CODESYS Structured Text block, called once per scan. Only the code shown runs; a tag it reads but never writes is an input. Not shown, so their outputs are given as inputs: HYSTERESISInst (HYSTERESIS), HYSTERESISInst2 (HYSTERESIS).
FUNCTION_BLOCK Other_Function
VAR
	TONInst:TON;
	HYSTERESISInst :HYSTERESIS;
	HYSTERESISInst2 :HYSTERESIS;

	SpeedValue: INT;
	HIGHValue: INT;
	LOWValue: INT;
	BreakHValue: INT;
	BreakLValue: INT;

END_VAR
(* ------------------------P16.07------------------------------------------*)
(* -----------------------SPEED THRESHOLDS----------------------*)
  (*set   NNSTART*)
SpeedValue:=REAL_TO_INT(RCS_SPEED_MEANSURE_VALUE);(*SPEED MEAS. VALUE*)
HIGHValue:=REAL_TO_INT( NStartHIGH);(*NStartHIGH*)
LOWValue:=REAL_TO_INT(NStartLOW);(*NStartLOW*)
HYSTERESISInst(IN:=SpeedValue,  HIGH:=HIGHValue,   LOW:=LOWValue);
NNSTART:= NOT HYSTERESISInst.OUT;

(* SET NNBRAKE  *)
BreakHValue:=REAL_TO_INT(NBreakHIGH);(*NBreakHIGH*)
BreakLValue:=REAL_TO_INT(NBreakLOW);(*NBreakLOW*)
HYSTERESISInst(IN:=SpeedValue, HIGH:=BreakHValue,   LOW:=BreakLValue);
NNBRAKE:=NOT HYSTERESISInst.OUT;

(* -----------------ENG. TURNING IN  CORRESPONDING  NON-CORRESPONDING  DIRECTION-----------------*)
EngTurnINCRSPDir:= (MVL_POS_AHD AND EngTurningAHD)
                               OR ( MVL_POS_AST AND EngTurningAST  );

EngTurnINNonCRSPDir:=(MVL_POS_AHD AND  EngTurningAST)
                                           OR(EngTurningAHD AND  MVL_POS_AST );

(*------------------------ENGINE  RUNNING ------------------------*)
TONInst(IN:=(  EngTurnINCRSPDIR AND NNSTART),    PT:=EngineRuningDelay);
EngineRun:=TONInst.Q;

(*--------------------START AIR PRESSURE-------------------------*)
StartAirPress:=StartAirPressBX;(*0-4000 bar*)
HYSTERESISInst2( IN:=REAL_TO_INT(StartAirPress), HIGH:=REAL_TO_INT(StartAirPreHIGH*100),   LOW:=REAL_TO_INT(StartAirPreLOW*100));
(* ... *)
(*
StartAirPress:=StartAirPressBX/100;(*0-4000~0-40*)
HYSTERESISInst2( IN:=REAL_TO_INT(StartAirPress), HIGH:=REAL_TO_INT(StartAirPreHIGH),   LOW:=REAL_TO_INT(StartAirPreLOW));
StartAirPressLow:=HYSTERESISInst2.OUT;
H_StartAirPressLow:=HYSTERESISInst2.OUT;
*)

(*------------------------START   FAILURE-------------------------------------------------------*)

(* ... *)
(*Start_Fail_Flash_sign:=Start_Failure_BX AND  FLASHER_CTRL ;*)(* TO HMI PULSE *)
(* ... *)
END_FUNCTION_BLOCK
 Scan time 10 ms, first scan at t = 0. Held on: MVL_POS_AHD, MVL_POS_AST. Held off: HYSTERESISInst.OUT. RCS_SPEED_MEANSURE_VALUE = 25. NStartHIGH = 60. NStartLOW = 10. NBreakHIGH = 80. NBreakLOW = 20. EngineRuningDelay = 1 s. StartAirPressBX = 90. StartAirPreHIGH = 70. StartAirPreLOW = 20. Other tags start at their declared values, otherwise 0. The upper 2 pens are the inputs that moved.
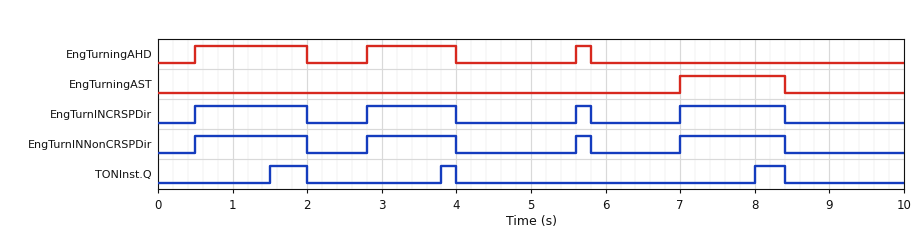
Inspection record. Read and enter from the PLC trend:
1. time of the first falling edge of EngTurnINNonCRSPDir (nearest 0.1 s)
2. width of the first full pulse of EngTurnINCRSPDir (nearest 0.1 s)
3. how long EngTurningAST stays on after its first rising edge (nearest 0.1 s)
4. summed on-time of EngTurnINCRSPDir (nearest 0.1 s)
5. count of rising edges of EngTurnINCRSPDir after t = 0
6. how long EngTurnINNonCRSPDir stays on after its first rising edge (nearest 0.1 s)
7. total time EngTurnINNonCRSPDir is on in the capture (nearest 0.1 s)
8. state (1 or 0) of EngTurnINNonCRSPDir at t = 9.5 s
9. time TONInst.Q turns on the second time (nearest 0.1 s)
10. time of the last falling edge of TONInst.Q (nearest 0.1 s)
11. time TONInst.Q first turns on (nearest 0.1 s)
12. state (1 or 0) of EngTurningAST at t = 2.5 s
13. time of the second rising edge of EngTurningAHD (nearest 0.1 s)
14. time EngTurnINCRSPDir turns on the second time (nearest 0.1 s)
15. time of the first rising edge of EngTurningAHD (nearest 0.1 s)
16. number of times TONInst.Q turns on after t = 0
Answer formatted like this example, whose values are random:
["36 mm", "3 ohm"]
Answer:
["2.0 s", "1.5 s", "1.4 s", "4.3 s", "4", "1.5 s", "4.3 s", "0", "3.8 s", "8.4 s", "1.5 s", "0", "2.8 s", "2.8 s", "0.5 s", "3"]
